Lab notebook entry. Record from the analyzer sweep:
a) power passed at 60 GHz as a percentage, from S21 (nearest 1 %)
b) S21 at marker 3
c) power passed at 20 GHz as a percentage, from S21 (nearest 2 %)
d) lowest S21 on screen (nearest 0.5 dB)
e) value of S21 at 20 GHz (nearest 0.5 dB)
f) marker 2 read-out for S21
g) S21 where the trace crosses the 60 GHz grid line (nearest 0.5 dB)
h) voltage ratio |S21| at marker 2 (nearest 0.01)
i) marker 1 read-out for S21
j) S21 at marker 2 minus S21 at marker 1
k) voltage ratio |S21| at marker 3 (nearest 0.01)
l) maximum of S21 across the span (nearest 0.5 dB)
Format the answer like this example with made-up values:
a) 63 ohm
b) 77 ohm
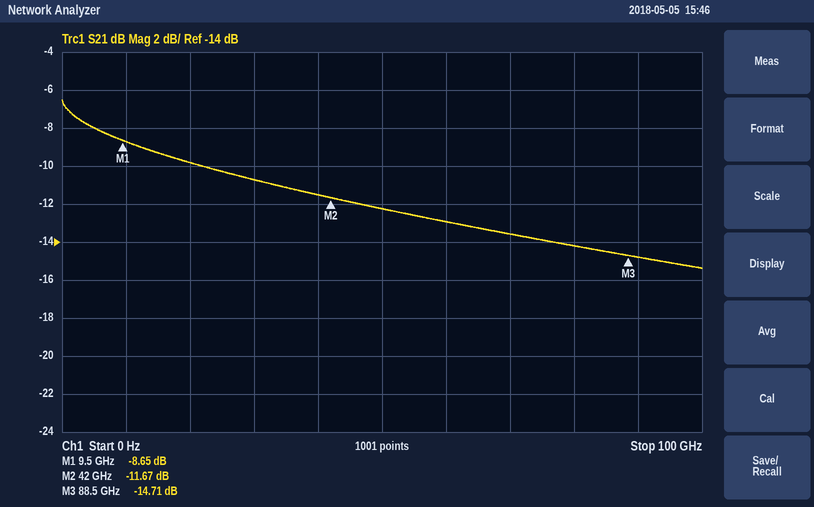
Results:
a) 5 %
b) -14.71 dB
c) 10 %
d) -15.5 dB
e) -10.0 dB
f) -11.67 dB
g) -13.0 dB
h) 0.26
i) -8.65 dB
j) -3.02 dB
k) 0.18
l) -6.5 dB
